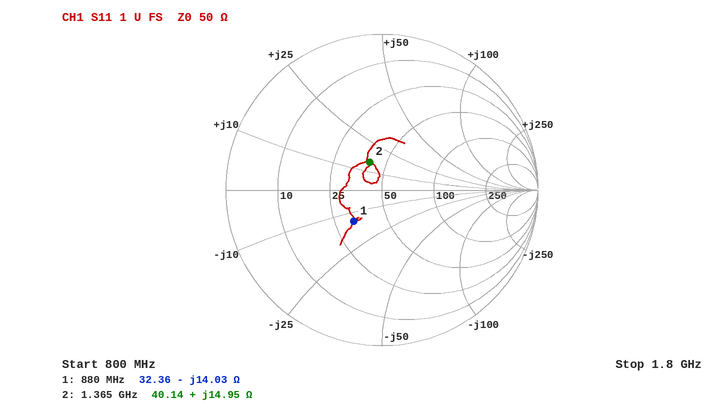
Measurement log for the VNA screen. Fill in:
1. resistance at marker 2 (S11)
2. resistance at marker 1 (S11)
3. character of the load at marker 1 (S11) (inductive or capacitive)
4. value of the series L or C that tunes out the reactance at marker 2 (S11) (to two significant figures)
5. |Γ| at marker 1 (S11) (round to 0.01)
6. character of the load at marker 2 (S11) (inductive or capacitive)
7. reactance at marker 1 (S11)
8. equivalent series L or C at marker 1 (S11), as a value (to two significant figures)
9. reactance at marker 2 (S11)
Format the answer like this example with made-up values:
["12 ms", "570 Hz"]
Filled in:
["40.14 Ω", "32.36 Ω", "capacitive", "7.8 pF", "0.27", "inductive", "-14.03 Ω", "13 pF", "+14.95 Ω"]
